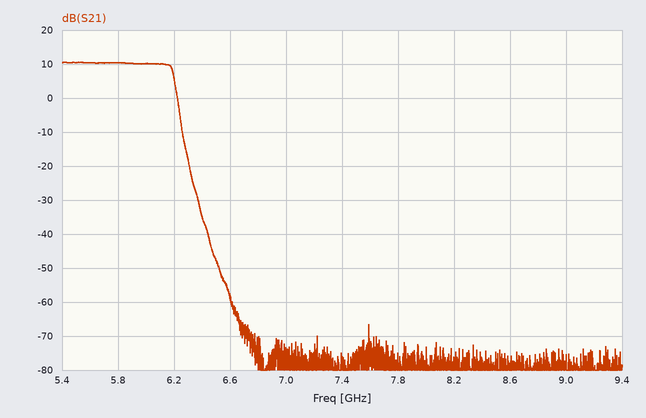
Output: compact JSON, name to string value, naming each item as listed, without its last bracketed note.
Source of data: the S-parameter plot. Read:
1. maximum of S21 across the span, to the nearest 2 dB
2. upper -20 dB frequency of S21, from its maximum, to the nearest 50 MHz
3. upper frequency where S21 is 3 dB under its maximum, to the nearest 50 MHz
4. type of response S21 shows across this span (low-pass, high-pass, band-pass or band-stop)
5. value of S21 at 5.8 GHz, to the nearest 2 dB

{"maximum of S21 across the span, to the nearest 2 dB": "10 dB", "upper -20 dB frequency of S21, from its maximum, to the nearest 50 MHz": "6.25 GHz", "upper frequency where S21 is 3 dB under its maximum, to the nearest 50 MHz": "6.20 GHz", "type of response S21 shows across this span": "low-pass", "value of S21 at 5.8 GHz, to the nearest 2 dB": "10 dB"}
